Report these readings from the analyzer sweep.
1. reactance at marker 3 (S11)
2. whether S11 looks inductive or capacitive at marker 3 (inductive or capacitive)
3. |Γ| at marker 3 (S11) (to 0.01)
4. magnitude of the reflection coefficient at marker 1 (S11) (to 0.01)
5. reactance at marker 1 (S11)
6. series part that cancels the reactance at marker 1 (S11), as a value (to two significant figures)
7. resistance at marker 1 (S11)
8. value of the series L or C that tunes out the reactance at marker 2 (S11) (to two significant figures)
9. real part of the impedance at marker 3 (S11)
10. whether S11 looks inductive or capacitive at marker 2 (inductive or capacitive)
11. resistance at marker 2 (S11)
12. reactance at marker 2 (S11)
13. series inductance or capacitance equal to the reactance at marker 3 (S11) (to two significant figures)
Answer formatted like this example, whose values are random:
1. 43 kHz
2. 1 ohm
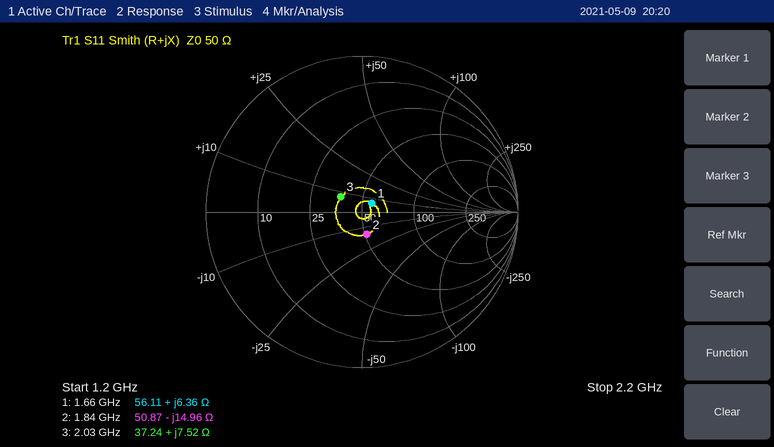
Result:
1. +7.52 Ω
2. inductive
3. 0.17
4. 0.08
5. +6.36 Ω
6. 15 pF
7. 56.11 Ω
8. 1.3 nH
9. 37.24 Ω
10. capacitive
11. 50.87 Ω
12. -14.96 Ω
13. 590 pH
